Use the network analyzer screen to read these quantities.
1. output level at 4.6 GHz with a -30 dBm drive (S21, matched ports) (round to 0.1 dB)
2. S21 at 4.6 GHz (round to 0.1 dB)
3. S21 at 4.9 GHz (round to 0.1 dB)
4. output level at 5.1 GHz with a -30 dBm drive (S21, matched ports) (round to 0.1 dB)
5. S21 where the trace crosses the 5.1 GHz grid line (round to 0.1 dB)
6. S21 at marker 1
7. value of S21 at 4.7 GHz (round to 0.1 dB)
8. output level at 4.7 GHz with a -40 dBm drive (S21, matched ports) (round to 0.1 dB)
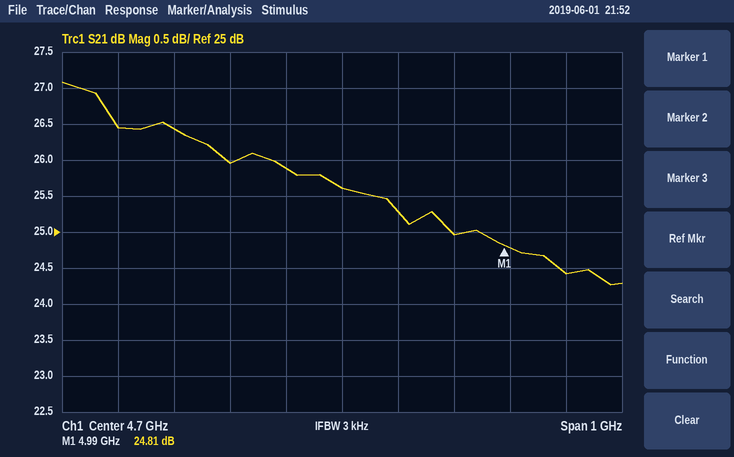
-4.1 dBm
25.9 dB
25.0 dB
-5.6 dBm
24.4 dB
24.81 dB
25.6 dB
-14.4 dBm
